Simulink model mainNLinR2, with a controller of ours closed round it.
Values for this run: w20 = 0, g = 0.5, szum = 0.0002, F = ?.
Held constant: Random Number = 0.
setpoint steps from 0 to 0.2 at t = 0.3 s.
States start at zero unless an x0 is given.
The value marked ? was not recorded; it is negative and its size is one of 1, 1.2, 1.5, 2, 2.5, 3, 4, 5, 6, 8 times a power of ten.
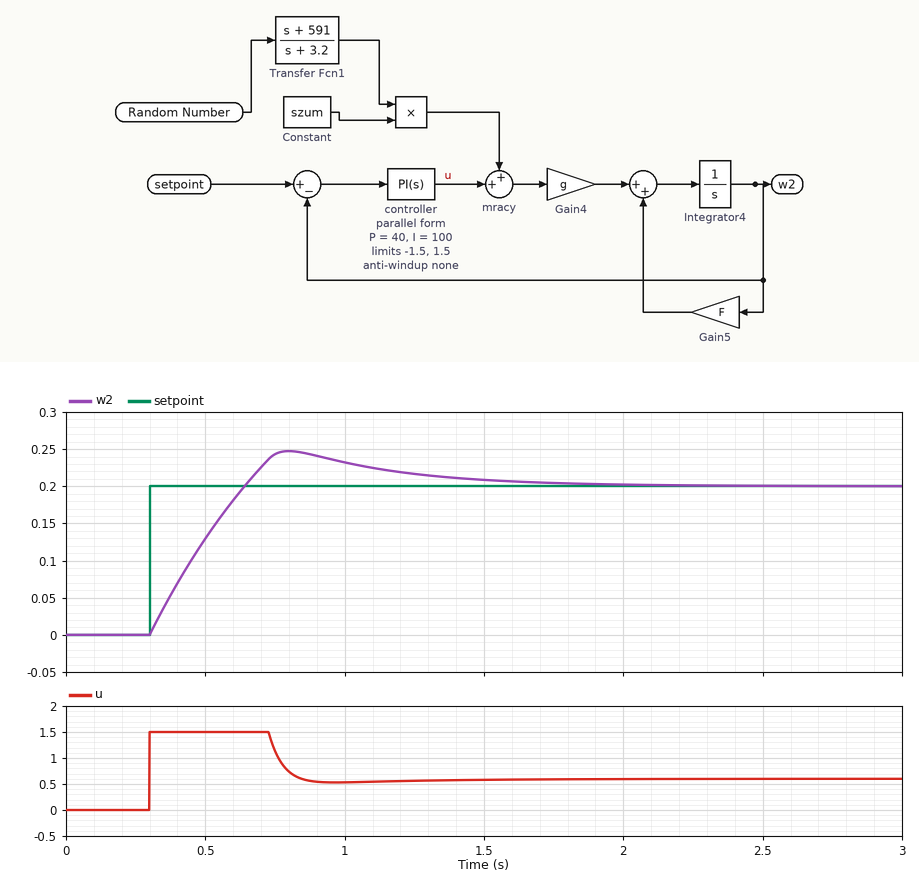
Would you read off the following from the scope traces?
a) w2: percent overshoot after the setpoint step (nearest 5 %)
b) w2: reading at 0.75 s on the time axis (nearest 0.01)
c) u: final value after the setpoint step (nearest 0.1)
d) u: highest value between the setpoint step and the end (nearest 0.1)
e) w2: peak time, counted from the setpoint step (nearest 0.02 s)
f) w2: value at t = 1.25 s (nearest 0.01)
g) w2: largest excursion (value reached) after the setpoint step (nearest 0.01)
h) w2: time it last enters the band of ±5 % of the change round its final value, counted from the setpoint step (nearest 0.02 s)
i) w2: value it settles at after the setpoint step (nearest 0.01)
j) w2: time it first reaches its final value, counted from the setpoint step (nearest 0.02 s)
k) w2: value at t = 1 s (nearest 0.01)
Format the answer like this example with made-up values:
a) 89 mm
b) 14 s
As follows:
a) 25 %
b) 0.24
c) 0.6
d) 1.5
e) 0.50 s
f) 0.22
g) 0.25
h) 1.14 s
i) 0.20
j) 0.34 s
k) 0.23
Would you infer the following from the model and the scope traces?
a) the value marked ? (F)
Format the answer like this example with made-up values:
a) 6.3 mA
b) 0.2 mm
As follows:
a) -1.5
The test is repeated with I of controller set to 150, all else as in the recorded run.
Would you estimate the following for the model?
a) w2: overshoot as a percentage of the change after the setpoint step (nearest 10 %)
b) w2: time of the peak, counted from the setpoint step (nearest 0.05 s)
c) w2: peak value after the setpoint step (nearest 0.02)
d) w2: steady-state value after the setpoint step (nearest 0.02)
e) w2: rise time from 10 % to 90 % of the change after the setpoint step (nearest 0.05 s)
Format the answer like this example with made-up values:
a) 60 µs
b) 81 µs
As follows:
a) 30 %
b) 0.55 s
c) 0.26
d) 0.20
e) 0.25 s
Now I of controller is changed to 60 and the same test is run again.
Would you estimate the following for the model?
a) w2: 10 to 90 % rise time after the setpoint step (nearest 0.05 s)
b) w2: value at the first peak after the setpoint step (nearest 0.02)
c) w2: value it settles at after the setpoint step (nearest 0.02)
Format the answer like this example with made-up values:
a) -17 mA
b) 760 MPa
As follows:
a) 0.25 s
b) 0.22
c) 0.20
